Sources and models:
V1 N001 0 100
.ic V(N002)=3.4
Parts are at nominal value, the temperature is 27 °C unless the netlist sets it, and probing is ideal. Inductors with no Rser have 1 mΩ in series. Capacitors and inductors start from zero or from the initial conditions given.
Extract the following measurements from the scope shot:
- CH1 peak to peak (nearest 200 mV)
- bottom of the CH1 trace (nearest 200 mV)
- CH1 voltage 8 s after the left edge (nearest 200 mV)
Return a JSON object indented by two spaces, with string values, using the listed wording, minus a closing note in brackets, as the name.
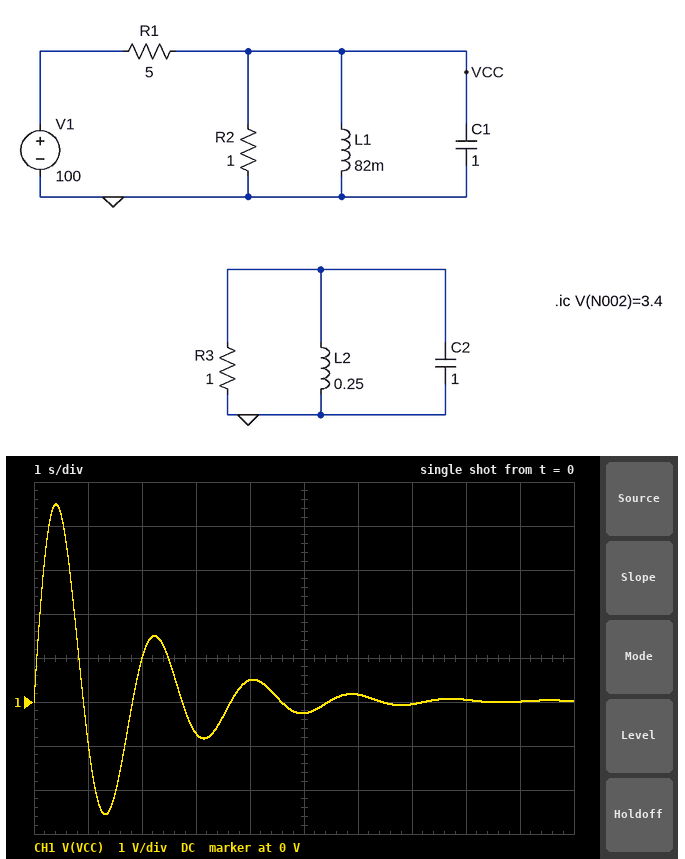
{
  "CH1 peak to peak": "7.0 V",
  "bottom of the CH1 trace": "-2.6 V",
  "CH1 voltage 8 s after the left edge": "0 V"
}
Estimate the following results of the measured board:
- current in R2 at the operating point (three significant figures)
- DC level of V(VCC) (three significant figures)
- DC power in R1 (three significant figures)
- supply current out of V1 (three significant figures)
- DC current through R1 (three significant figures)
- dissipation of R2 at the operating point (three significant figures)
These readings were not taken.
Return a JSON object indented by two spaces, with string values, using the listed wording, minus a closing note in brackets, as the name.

{
  "current in R2 at the operating point": "20.0 mA",
  "DC level of V(VCC)": "20.0 mV",
  "DC power in R1": "2.00 kW",
  "supply current out of V1": "20.0 A",
  "DC current through R1": "20.0 A",
  "dissipation of R2 at the operating point": "399 µW"
}
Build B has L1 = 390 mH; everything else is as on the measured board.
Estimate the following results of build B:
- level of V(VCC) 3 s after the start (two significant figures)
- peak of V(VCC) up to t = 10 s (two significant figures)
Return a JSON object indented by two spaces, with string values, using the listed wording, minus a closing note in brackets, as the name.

{
  "level of V(VCC) 3 s after the start": "-2.1 V",
  "peak of V(VCC) up to t = 10 s": "7.7 V"
}
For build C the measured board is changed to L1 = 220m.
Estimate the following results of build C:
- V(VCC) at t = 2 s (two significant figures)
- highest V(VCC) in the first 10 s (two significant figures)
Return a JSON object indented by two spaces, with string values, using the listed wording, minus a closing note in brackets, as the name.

{
  "V(VCC) at t = 2 s": "-2.4 V",
  "highest V(VCC) in the first 10 s": "6.4 V"
}
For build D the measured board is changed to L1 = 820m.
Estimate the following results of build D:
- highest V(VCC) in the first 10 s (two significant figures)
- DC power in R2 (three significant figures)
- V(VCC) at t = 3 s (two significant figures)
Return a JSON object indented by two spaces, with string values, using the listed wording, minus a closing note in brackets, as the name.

{
  "highest V(VCC) in the first 10 s": "9.5 V",
  "DC power in R2": "399 µW",
  "V(VCC) at t = 3 s": "1.3 V"
}
